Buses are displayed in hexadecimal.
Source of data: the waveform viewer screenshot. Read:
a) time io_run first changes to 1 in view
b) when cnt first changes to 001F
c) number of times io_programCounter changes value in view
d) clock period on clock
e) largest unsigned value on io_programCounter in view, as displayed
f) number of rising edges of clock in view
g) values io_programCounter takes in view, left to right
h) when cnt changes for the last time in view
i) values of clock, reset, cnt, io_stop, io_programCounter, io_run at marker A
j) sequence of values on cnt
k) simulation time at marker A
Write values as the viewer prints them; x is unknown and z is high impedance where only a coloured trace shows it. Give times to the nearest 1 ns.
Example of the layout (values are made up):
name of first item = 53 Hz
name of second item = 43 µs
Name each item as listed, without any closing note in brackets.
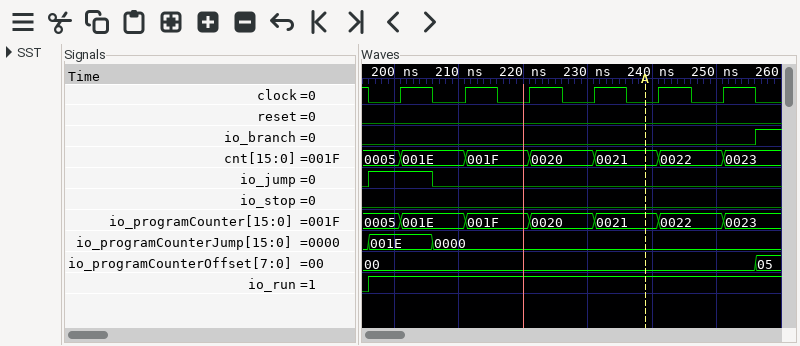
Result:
time io_run first changes to 1 in view = 196 ns
when cnt first changes to 001F = 211 ns
number of times io_programCounter changes value in view = 6
clock period on clock = 10 ns
largest unsigned value on io_programCounter in view, as displayed = 0023
number of rising edges of clock in view = 6
values io_programCounter takes in view, left to right = 0005, 001E, 001F, 0020, 0021, 0022, 0023
when cnt changes for the last time in view = 251 ns
values of clock, reset, cnt, io_stop, io_programCounter, io_run at marker A = clock=0, reset=0, cnt=0021, io_stop=0, io_programCounter=0021, io_run=1
sequence of values on cnt = 0005, 001E, 001F, 0020, 0021, 0022, 0023
simulation time at marker A = 239 ns
